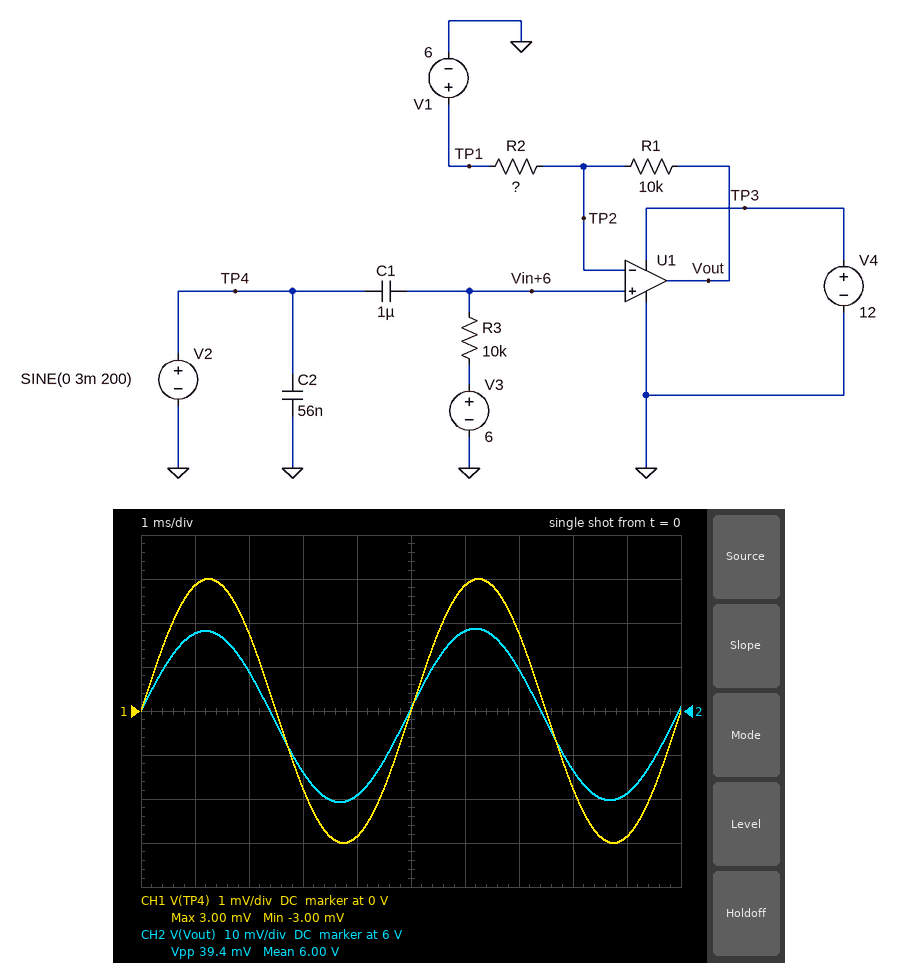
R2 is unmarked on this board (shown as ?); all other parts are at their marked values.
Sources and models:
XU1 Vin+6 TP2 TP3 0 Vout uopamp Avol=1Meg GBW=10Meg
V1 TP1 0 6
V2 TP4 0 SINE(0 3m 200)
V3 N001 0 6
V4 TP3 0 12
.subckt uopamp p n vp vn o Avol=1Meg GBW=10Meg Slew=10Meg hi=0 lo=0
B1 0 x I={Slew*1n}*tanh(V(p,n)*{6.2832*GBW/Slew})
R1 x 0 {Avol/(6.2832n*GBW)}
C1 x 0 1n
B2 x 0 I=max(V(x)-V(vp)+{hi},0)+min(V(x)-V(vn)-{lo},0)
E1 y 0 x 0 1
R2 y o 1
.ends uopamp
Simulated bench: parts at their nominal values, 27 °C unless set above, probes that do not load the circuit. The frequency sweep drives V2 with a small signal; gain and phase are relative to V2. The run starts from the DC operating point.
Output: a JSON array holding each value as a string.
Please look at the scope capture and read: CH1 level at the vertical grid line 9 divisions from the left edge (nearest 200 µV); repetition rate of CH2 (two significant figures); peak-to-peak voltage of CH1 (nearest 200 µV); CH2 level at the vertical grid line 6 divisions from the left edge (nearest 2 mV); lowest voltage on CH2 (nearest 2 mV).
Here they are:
["-2.8 mV", "200 Hz", "6.0 mV", "6.018 V", "5.980 V"]
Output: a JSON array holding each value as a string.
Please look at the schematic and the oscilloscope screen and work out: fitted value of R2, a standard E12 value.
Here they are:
["1.8 kΩ"]
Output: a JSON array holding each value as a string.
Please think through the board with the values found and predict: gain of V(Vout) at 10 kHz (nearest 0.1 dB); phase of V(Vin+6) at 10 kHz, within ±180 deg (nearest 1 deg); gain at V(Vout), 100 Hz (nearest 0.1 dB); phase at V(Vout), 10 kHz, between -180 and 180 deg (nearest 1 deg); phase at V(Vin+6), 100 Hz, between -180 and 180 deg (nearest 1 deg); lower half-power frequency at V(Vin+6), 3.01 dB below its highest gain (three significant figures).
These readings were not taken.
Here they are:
["16.3 dB", "0 deg", "16.2 dB", "0 deg", "9 deg", "15.9 Hz"]
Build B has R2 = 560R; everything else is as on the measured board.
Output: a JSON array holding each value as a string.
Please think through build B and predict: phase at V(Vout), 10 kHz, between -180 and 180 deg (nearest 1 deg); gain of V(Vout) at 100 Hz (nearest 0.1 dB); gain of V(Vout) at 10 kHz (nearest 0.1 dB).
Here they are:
["-1 deg", "25.4 dB", "25.5 dB"]
